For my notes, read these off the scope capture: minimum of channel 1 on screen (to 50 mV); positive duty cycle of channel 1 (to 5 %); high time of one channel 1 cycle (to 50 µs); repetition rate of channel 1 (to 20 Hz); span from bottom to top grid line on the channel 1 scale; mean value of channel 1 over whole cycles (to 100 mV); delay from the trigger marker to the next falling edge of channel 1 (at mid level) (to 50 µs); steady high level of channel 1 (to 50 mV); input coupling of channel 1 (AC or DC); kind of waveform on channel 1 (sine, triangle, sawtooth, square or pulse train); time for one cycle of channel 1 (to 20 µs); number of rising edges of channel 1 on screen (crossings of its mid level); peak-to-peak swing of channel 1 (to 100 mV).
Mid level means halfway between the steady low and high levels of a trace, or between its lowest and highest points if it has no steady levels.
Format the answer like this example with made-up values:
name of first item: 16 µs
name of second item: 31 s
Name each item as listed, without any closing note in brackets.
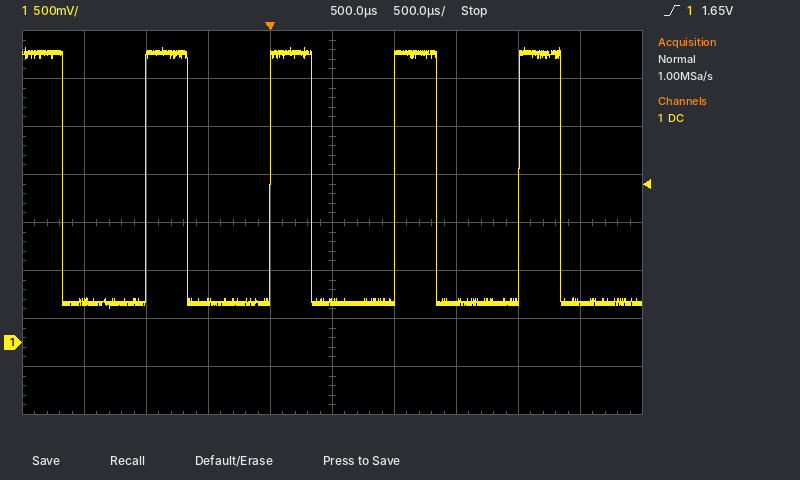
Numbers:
minimum of channel 1 on screen: 350 mV
positive duty cycle of channel 1: 35 %
high time of one channel 1 cycle: 350 µs
repetition rate of channel 1: 1.00 kHz
span from bottom to top grid line on the channel 1 scale: 4 V
mean value of channel 1 over whole cycles: 1.3 V
delay from the trigger marker to the next falling edge of channel 1 (at mid level): 350 µs
steady high level of channel 1: 3.00 V
input coupling of channel 1: DC
kind of waveform on channel 1: pulse train
time for one cycle of channel 1: 1.00 ms
number of rising edges of channel 1 on screen: 4
peak-to-peak swing of channel 1: 2.70 V
